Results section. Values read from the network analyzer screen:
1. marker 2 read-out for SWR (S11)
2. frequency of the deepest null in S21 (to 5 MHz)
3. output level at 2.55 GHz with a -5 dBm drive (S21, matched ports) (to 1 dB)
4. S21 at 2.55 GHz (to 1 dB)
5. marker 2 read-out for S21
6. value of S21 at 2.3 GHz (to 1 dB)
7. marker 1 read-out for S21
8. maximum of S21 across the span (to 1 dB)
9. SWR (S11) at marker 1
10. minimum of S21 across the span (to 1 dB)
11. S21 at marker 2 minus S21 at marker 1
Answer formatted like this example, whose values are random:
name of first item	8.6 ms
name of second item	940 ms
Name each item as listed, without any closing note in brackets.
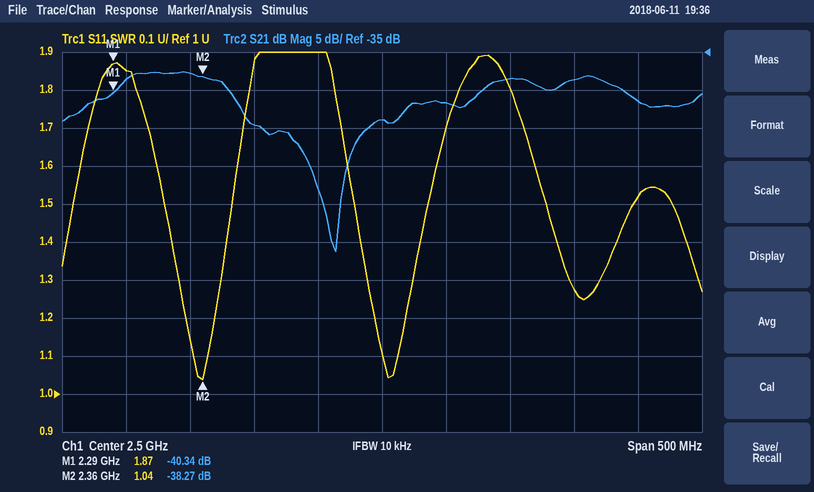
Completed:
marker 2 read-out for SWR	1.04
frequency of the deepest null in S21	2.465 GHz
output level at 2.55 GHz with a -5 dBm drive (S21, matched ports)	-47 dBm
S21 at 2.55 GHz	-42 dB
marker 2 read-out for S21	-38.27 dB
value of S21 at 2.3 GHz	-39 dB
marker 1 read-out for S21	-40.34 dB
maximum of S21 across the span	-38 dB
SWR (S11) at marker 1	1.87
minimum of S21 across the span	-61 dB
S21 at marker 2 minus S21 at marker 1	2.07 dB
